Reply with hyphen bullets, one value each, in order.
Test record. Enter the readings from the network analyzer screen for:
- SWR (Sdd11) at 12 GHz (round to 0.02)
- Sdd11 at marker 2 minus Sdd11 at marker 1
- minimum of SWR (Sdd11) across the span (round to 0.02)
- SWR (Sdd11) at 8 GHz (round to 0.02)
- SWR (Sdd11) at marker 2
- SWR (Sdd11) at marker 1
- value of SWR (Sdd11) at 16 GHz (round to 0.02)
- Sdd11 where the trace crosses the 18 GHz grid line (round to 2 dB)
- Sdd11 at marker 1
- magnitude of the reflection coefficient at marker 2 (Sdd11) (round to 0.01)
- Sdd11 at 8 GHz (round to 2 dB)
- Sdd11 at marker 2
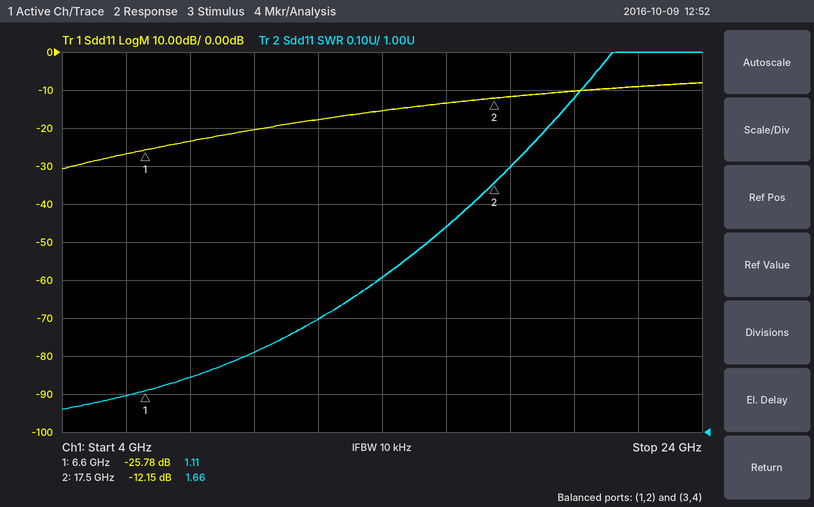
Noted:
- 1.30
- 13.63 dB
- 1.06
- 1.14
- 1.66
- 1.11
- 1.54
- -12 dB
- -25.78 dB
- 0.25
- -24 dB
- -12.15 dB
